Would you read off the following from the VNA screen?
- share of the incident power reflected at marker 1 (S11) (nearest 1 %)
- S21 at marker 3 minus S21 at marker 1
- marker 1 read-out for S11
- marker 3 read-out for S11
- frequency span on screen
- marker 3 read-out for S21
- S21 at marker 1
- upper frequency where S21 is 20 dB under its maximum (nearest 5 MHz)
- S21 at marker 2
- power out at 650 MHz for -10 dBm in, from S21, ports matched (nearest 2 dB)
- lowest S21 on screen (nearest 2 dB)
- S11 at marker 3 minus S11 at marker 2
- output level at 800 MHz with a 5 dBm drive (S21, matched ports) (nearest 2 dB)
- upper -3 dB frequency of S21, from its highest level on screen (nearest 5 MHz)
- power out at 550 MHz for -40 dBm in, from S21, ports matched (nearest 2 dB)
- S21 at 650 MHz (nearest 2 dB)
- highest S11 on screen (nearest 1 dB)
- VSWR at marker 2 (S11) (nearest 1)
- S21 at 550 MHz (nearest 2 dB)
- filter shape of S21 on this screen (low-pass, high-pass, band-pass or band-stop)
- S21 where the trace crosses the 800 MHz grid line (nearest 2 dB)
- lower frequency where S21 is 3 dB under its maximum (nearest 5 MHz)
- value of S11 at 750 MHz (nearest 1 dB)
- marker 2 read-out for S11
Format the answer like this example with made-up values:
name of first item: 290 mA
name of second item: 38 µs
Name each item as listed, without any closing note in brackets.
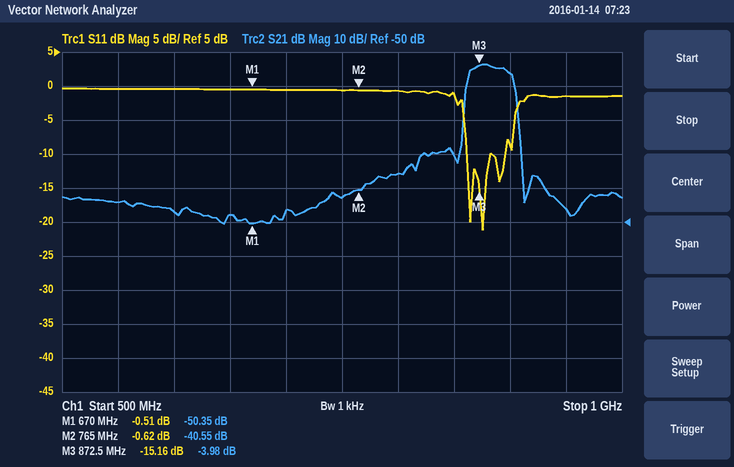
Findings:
share of the incident power reflected at marker 1 (S11): 89 %
S21 at marker 3 minus S21 at marker 1: 46.37 dB
marker 1 read-out for S11: -0.51 dB
marker 3 read-out for S11: -15.16 dB
frequency span on screen: 500 MHz
marker 3 read-out for S21: -3.98 dB
S21 at marker 1: -50.35 dB
upper frequency where S21 is 20 dB under its maximum: 910 MHz
S21 at marker 2: -40.55 dB
power out at 650 MHz for -10 dBm in, from S21, ports matched: -58 dBm
lowest S21 on screen: -50 dB
S11 at marker 3 minus S11 at marker 2: -14.54 dB
output level at 800 MHz with a 5 dBm drive (S21, matched ports): -30 dBm
upper -3 dB frequency of S21, from its highest level on screen: 900 MHz
power out at 550 MHz for -40 dBm in, from S21, ports matched: -84 dBm
S21 at 650 MHz: -48 dB
highest S11 on screen: 0 dB
VSWR at marker 2 (S11): 28
S21 at 550 MHz: -44 dB
filter shape of S21 on this screen: band-pass
S21 where the trace crosses the 800 MHz grid line: -36 dB
lower frequency where S21 is 3 dB under its maximum: 865 MHz
value of S11 at 750 MHz: -1 dB
marker 2 read-out for S11: -0.62 dB
